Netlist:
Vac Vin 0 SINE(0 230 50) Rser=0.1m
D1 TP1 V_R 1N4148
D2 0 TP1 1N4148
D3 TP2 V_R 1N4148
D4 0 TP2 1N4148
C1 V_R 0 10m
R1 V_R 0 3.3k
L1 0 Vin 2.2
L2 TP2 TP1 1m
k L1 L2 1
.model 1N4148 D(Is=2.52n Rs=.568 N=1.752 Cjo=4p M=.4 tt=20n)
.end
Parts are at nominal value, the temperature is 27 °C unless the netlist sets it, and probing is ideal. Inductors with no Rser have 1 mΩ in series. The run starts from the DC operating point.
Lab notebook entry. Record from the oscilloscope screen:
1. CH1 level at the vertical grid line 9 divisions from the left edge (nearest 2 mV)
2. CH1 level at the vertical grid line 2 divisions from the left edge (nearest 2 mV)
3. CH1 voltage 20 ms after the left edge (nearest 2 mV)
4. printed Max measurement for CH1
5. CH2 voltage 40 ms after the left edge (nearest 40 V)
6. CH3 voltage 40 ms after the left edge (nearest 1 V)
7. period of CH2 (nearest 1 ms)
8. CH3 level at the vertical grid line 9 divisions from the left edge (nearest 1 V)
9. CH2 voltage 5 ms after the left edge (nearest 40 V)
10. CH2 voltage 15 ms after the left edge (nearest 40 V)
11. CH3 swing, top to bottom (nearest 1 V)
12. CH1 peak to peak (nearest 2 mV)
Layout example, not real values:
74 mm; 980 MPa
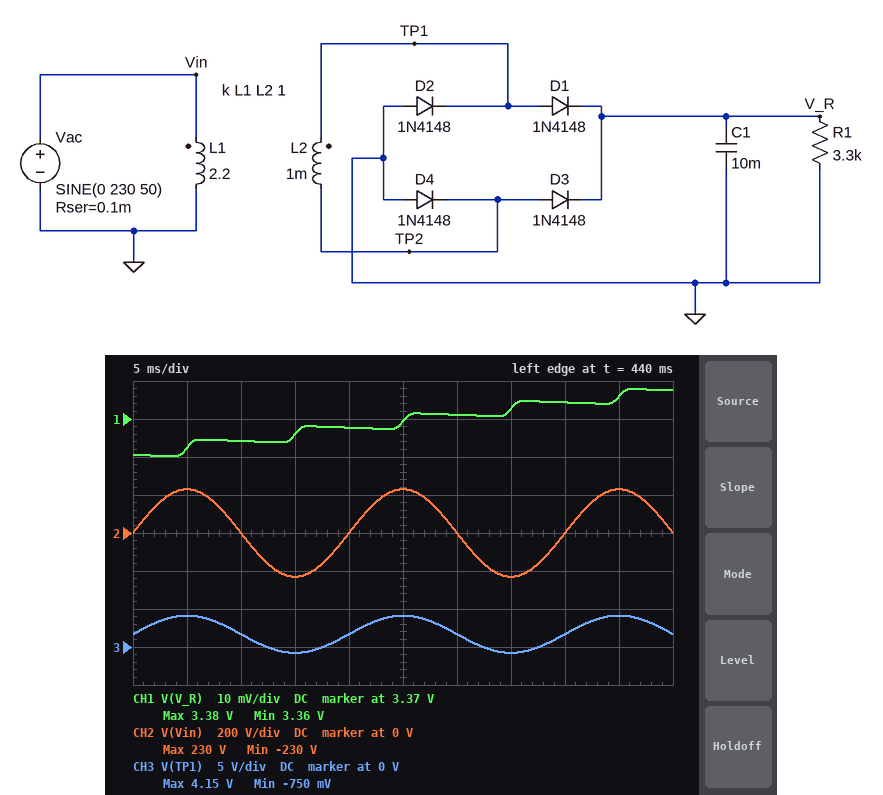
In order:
3.376 V; 3.364 V; 3.368 V; 3.38 V; 0 V; 2 V; 20 ms; 4 V; 240 V; -240 V; 5 V; 18 mV
